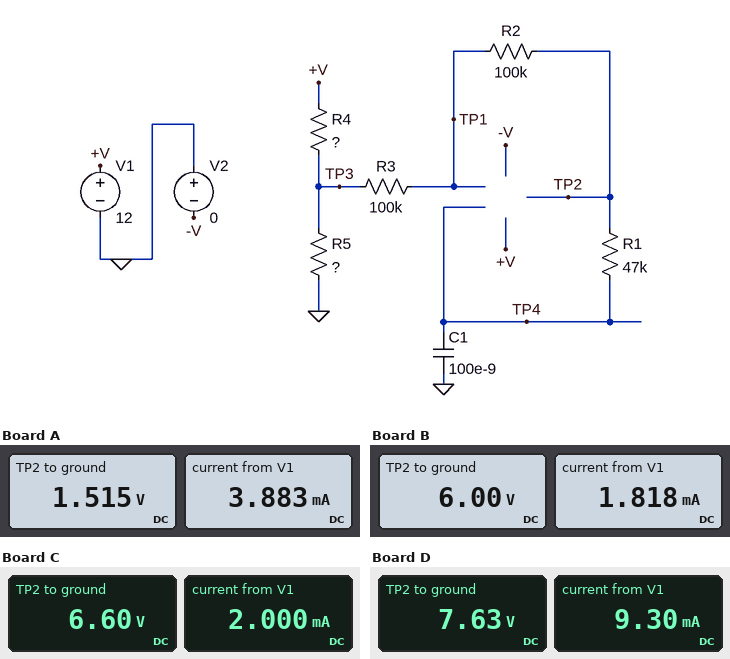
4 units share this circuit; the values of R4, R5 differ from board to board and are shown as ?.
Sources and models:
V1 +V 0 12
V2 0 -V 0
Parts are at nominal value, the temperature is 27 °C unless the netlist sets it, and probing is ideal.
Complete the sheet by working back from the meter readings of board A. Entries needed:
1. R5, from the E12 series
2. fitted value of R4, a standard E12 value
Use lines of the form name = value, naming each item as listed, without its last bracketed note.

R5, from the E12 series = 390 Ω
fitted value of R4, a standard E12 value = 2.7 kΩ
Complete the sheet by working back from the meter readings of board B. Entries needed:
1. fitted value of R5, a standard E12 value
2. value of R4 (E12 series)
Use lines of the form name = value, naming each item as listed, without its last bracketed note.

fitted value of R5, a standard E12 value = 3.3 kΩ
value of R4 = 3.3 kΩ
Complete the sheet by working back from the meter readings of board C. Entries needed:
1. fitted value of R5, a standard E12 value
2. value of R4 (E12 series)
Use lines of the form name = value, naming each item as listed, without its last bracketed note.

fitted value of R5, a standard E12 value = 3.3 kΩ
value of R4 = 2.7 kΩ
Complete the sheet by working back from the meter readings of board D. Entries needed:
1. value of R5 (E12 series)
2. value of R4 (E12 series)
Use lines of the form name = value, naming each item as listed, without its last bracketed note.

value of R5 = 820 Ω
value of R4 = 470 Ω
